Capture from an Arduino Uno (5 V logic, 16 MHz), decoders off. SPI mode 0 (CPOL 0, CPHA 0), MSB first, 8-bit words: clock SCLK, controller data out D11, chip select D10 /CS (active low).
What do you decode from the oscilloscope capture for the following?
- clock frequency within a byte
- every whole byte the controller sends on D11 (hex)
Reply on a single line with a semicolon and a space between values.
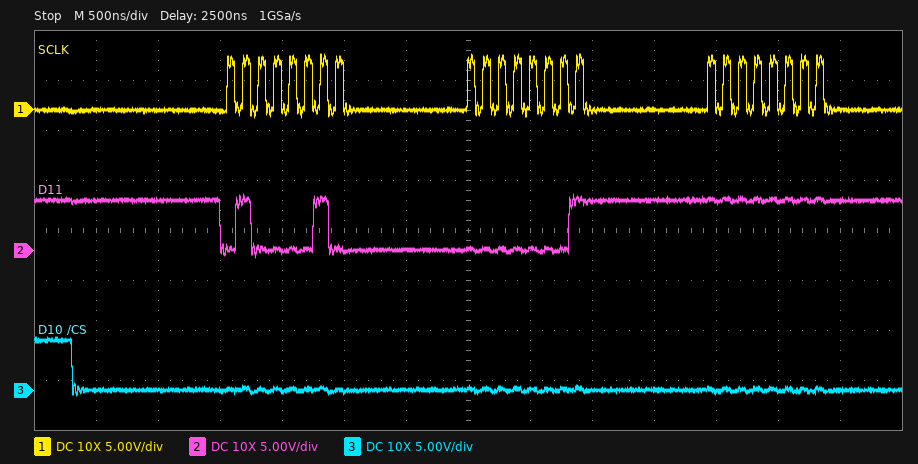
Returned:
8 MHz; 42 01 FF
